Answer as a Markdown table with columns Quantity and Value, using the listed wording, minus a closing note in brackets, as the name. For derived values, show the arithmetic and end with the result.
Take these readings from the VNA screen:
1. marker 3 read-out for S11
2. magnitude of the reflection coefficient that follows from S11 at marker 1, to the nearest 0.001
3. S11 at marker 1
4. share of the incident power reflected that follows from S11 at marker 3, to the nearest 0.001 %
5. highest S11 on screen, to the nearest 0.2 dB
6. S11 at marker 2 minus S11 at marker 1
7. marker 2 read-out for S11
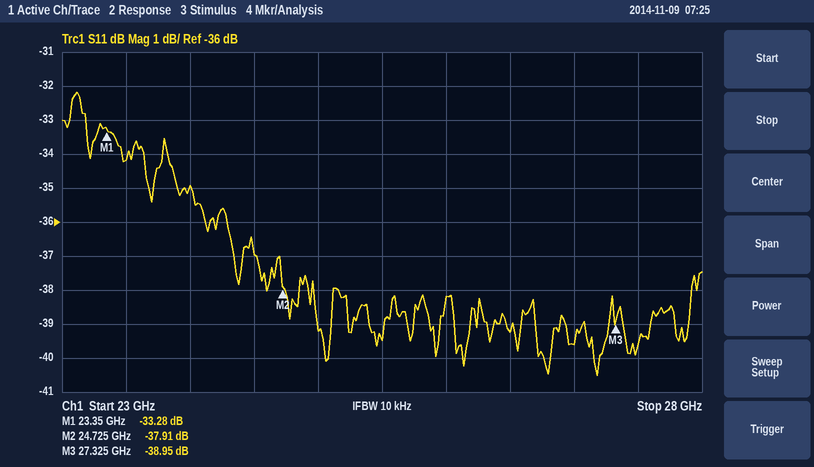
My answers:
| Quantity | Value |
|---|---|
| marker 3 read-out for S11 | -38.95 dB |
| magnitude of the reflection coefficient that follows from S11 at marker 1, to the nearest 0.001 | 10^(-33.28/20) ≈ 0.022 |
| S11 at marker 1 | -33.28 dB |
| share of the incident power reflected that follows from S11 at marker 3, to the nearest 0.001 % | 10^(-38.95/10) ≈ 0.013 % |
| highest S11 on screen, to the nearest 0.2 dB | -32.2 dB |
| S11 at marker 2 minus S11 at marker 1 | -37.91 − (-33.28) = -4.63 dB |
| marker 2 read-out for S11 | -37.91 dB |
